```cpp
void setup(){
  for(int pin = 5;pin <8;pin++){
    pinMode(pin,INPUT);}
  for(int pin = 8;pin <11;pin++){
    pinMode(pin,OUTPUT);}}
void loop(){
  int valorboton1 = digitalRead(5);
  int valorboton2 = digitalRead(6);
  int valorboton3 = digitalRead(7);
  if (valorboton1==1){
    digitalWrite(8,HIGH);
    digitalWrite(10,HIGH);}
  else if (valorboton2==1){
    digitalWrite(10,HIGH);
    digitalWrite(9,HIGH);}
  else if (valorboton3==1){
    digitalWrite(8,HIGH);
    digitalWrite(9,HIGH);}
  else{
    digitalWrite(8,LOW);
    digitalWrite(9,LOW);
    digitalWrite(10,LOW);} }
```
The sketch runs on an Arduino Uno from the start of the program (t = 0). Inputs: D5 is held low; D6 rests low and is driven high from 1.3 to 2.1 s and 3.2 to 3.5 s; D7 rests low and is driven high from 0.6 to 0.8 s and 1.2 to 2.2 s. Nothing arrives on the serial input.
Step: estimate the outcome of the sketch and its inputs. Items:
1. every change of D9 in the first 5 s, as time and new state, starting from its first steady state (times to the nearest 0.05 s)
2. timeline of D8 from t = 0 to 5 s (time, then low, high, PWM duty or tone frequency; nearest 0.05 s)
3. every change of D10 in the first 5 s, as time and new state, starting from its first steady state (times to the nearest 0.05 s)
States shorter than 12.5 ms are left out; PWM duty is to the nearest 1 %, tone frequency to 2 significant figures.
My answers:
0 s low; 0.6 s high; 0.8 s low; 1.2 s high; 2.2 s low; 3.2 s high; 3.5 s low
0 s low; 0.6 s high; 0.8 s low; 1.2 s high; 2.2 s low
0 s low; 1.3 s high; 2.2 s low; 3.2 s high; 3.5 s low
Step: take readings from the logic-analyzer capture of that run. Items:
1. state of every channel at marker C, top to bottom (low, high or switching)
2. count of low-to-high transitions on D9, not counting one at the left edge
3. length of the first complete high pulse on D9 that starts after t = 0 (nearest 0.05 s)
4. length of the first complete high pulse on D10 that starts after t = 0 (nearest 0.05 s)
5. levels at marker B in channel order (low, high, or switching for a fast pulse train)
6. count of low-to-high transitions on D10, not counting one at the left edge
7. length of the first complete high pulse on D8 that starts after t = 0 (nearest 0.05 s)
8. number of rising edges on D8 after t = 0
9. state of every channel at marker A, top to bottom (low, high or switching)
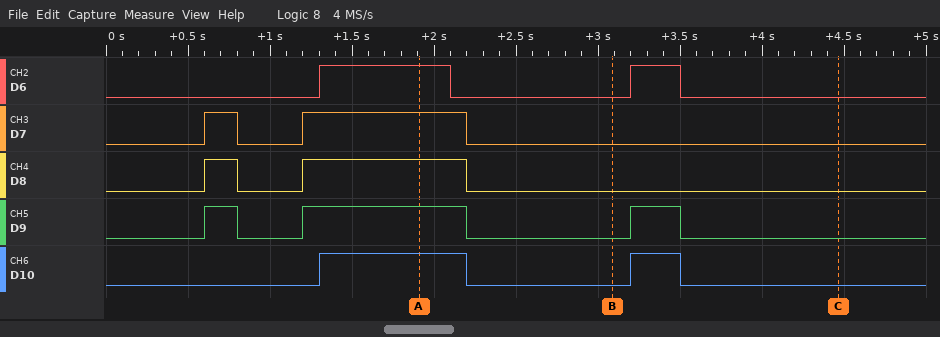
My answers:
D6 low, D7 low, D8 low, D9 low, D10 low
3
0.20 s
0.90 s
D6 low, D7 low, D8 low, D9 low, D10 low
2
0.20 s
2
D6 high, D7 high, D8 high, D9 high, D10 high
